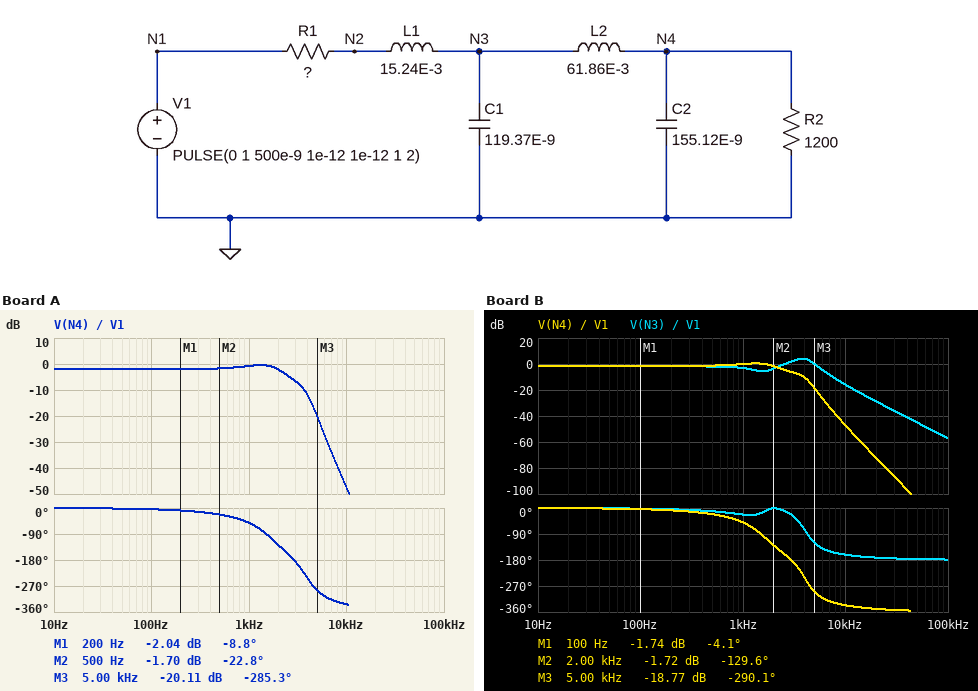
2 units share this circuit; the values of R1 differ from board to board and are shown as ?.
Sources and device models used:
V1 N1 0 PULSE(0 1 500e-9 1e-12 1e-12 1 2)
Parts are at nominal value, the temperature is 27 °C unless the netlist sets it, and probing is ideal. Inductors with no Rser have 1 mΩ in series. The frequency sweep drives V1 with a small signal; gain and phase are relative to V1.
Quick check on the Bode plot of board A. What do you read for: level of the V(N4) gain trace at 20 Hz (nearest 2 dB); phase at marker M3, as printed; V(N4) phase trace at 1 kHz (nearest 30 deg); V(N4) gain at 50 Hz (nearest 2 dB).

-2 dB
-285.3 deg
-60 deg
-2 dB
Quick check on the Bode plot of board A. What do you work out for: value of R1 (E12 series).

330 Ω
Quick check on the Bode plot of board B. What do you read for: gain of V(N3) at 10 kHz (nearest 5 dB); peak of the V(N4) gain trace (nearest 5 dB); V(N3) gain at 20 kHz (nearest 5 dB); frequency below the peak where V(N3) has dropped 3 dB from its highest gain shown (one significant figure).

-15 dB
0 dB
-30 dB
3 kHz
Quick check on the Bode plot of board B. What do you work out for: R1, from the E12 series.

270 Ω
